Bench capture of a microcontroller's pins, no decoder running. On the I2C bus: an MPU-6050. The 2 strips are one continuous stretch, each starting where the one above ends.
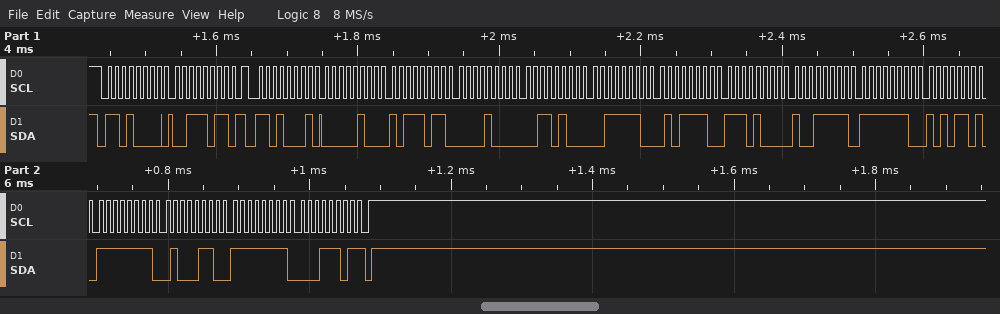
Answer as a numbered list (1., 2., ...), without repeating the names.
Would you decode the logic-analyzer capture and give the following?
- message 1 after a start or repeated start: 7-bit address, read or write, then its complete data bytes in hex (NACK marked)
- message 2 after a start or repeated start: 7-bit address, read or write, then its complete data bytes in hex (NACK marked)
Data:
1. 0x68 write: 3B
2. 0x68 read: 04 BB 08 34 3E 5E E8 9F FE AD FF 46 FF 1D NACK
